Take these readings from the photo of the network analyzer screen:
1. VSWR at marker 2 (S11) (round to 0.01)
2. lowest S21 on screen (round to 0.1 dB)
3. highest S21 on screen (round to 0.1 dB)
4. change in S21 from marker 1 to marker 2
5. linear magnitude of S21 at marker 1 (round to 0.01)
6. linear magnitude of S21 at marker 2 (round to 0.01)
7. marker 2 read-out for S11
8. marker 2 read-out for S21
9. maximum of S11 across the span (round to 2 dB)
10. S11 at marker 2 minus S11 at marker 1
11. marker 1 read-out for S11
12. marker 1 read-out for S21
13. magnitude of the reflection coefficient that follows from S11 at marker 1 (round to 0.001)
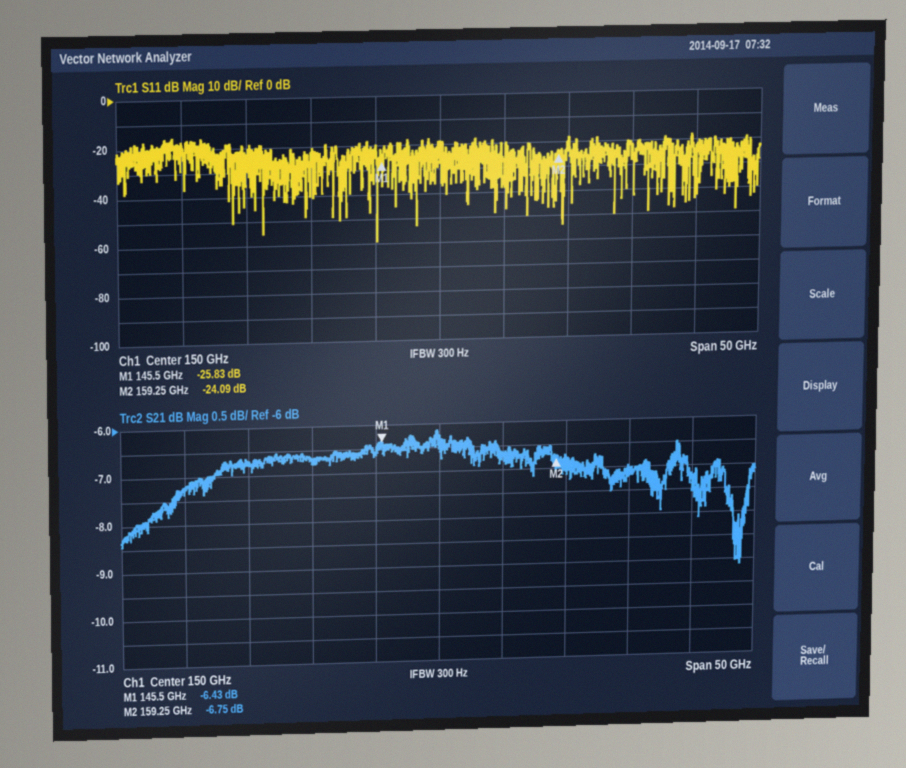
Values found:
1.13
-9.1 dB
-6.1 dB
-0.32 dB
0.48
0.46
-24.09 dB
-6.75 dB
-16 dB
1.74 dB
-25.83 dB
-6.43 dB
0.051
